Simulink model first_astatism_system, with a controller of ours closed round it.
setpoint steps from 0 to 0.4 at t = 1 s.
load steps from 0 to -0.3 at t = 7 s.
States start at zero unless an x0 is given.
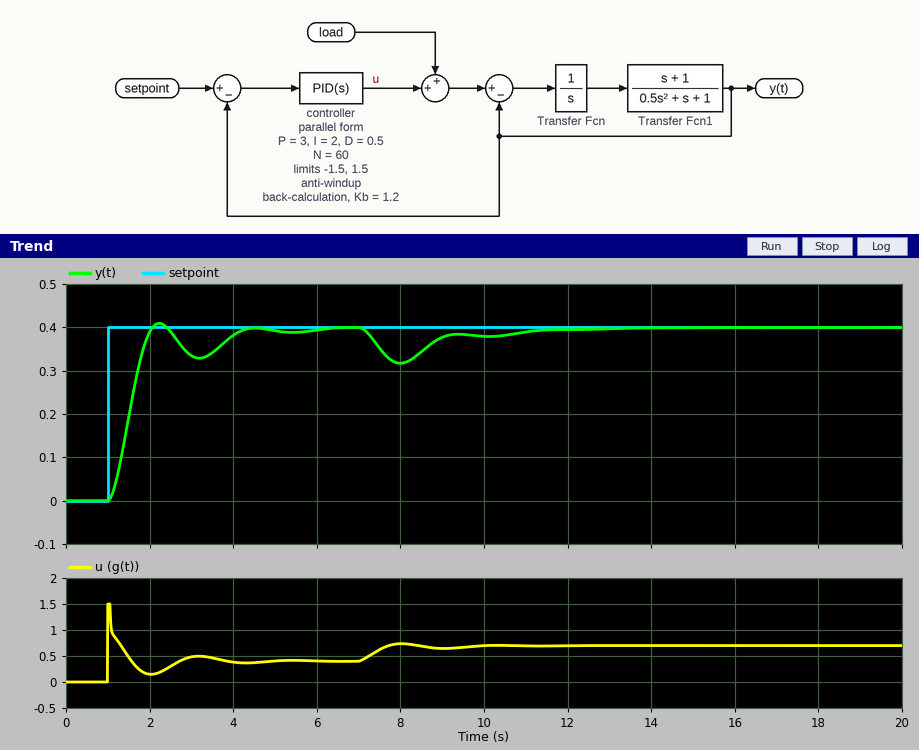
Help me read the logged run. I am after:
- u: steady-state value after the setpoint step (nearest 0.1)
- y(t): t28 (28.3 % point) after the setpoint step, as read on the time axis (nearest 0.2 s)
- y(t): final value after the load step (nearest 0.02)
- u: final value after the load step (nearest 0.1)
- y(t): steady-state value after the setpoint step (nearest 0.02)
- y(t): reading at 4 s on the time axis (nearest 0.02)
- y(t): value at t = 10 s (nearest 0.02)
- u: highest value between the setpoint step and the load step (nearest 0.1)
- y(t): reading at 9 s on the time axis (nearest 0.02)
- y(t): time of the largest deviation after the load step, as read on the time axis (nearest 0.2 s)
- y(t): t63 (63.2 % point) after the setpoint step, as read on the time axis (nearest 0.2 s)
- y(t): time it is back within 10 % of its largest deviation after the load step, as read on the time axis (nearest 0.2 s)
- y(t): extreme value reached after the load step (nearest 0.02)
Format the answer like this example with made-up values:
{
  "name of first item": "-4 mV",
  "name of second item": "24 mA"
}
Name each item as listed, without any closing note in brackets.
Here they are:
{
  "u: steady-state value after the setpoint step": "0.4",
  "y(t): t28 (28.3 % point) after the setpoint step, as read on the time axis": "1.4 s",
  "y(t): final value after the load step": "0.40",
  "u: final value after the load step": "0.7",
  "y(t): steady-state value after the setpoint step": "0.40",
  "y(t): reading at 4 s on the time axis": "0.38",
  "y(t): value at t = 10 s": "0.38",
  "u: highest value between the setpoint step and the load step": "1.5",
  "y(t): reading at 9 s on the time axis": "0.38",
  "y(t): time of the largest deviation after the load step, as read on the time axis": "8.0 s",
  "y(t): t63 (63.2 % point) after the setpoint step, as read on the time axis": "1.6 s",
  "y(t): time it is back within 10 % of its largest deviation after the load step, as read on the time axis": "11.2 s",
  "y(t): extreme value reached after the load step": "0.32"
}
